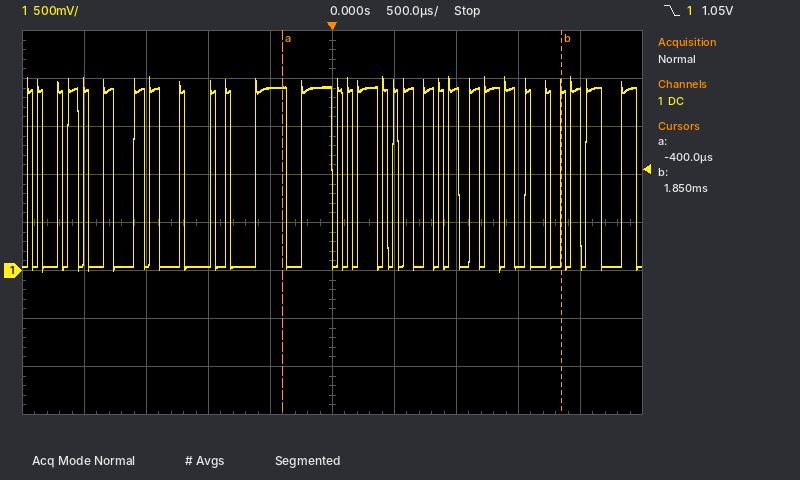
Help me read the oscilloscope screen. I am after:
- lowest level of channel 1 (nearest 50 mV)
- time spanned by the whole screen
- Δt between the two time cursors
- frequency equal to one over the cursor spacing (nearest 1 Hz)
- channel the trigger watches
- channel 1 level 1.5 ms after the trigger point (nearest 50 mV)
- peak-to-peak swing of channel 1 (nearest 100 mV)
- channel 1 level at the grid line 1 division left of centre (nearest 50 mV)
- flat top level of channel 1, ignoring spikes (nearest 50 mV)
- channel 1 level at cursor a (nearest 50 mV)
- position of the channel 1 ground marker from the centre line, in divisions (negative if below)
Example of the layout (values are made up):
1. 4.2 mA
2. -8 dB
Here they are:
1. 0 mV
2. 5 ms
3. 2.25 ms
4. 444 Hz
5. channel 1
6. 50 mV
7. 2.00 V
8. 1.90 V
9. 1.90 V
10. 1.90 V
11. -1.0 div
